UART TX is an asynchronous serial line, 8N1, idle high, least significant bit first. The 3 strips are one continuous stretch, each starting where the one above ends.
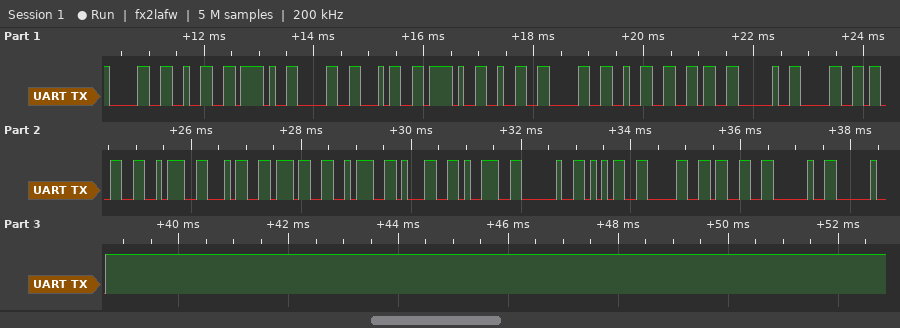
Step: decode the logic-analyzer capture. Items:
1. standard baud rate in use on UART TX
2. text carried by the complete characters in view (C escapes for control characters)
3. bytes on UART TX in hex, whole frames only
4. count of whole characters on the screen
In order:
9600 baud
"02/04/2026 03:47:19 503  "
30 32 2F 30 34 2F 32 30 32 36 20 30 33 3A 34 37 3A 31 39 20 35 30 33 20 20
25
